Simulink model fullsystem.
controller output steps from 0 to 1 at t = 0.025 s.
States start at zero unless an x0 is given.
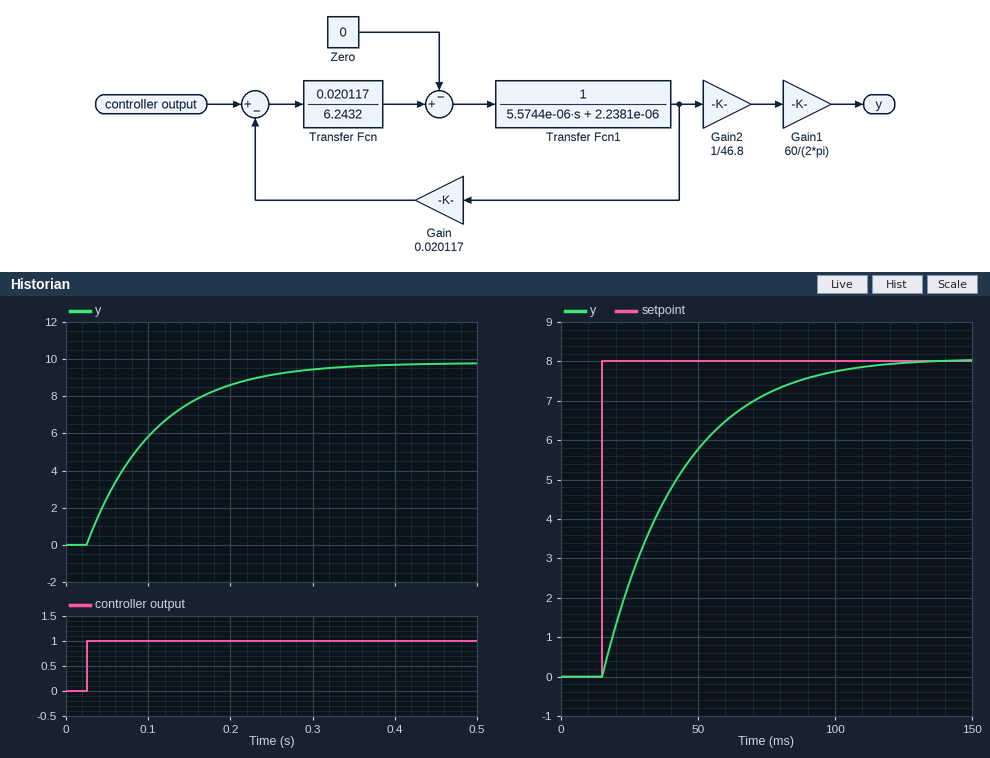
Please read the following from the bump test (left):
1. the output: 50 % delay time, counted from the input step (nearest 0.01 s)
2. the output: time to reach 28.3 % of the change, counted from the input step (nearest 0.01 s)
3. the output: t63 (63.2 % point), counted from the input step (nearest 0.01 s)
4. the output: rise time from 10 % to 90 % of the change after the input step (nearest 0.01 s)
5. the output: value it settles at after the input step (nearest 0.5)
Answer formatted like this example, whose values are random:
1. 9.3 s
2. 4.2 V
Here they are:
1. 0.06 s
2. 0.03 s
3. 0.08 s
4. 0.18 s
5. 10.0
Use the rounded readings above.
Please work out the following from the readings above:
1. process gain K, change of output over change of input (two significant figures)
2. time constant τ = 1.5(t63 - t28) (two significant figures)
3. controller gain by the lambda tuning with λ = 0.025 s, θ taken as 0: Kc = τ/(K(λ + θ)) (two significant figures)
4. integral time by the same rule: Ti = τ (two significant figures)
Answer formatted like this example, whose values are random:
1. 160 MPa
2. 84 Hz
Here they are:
1. 10
2. 0.075 s
3. 0.30
4. 0.075 s
